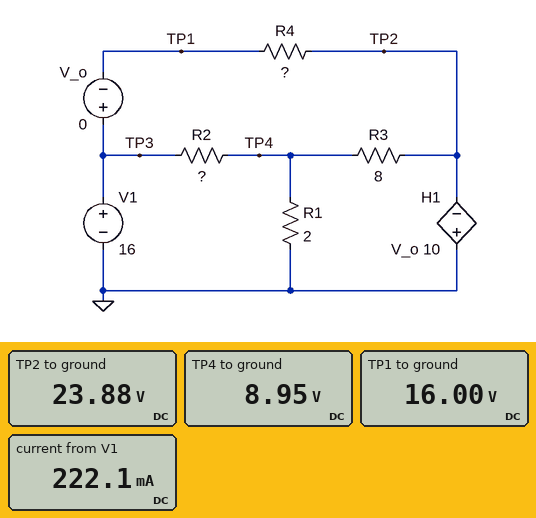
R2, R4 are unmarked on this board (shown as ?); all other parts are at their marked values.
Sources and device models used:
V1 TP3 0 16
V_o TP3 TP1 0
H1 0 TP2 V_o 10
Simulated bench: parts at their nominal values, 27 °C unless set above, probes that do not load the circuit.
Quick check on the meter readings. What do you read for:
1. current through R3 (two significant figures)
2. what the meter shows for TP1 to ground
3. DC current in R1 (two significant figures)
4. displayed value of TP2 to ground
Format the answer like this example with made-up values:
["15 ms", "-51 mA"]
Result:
["1.9 A", "16.00 V", "4.5 A", "23.88 V"]
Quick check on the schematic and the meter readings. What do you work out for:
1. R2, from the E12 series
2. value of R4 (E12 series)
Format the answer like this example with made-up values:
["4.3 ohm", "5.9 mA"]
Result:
["2.7 Ω", "3.3 Ω"]
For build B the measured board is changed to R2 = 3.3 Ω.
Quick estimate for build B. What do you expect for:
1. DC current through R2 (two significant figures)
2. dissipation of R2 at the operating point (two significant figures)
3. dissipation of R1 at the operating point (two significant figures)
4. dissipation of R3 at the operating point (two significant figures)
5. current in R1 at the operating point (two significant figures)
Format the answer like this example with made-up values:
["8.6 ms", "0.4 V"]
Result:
["2.3 A", "17 W", "36 W", "30 W", "4.2 A"]
